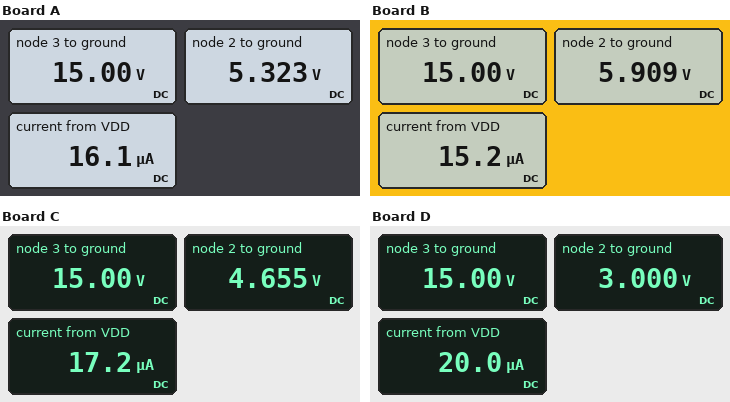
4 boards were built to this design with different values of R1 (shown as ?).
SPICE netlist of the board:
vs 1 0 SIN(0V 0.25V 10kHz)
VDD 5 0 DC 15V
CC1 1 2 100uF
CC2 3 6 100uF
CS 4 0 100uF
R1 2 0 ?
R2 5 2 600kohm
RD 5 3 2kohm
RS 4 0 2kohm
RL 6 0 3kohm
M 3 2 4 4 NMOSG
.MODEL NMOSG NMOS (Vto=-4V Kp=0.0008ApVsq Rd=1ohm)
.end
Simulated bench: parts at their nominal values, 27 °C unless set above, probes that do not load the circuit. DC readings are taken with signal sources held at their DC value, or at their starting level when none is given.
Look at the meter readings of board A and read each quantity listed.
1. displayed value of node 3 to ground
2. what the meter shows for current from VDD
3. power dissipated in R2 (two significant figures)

15.00 V
16.1 µA
160 µW
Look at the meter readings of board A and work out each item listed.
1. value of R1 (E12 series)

330 kΩ
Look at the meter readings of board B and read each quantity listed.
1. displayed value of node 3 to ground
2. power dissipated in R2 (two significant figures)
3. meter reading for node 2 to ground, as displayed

15.00 V
140 µW
5.909 V
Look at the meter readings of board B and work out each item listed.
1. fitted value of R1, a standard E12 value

390 kΩ
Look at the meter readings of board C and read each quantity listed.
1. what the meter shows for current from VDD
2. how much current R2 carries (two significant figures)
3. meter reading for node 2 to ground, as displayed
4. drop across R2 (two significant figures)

17.2 µA
17 µA
4.655 V
10 V
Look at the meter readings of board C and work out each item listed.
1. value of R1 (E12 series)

270 kΩ
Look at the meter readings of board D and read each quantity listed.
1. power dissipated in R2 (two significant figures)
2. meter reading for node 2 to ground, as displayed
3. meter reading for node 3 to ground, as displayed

240 µW
3.000 V
15.00 V
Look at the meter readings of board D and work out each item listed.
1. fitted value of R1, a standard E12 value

150 kΩ
